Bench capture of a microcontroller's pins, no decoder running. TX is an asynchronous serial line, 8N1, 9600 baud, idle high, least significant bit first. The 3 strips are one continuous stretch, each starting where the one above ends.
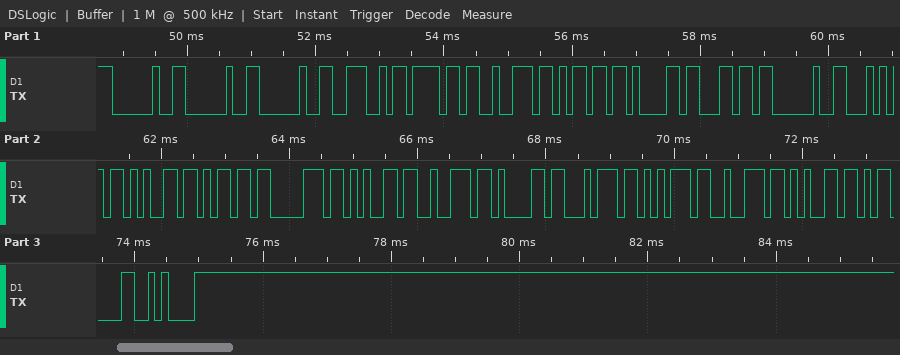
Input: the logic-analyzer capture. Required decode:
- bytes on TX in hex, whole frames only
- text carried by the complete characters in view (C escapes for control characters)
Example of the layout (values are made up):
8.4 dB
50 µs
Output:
0x20 0x20 0x20 0x4E 0x6F 0x72 0x6D 0x61 0x6C 0x20 0x54 0x65 0x6D 0x70 0x65 0x72 0x61 0x74 0x75 0x72 0x65 0x0D 0x0A
"   Normal Temperature\r\n"
